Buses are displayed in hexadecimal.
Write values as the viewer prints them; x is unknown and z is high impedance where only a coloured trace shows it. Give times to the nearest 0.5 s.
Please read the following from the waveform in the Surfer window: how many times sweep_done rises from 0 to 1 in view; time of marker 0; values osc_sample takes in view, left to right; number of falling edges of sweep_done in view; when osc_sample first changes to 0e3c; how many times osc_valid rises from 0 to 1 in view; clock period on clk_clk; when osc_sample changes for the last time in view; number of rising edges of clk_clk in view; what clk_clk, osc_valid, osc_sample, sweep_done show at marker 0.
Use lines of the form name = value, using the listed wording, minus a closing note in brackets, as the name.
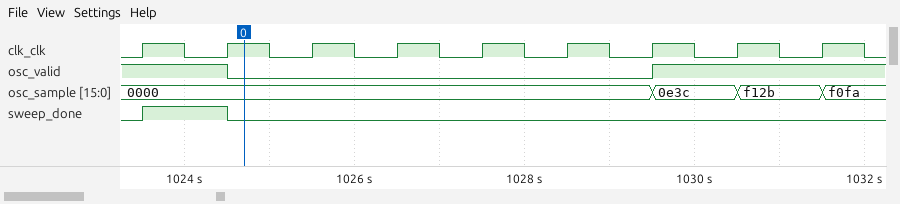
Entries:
how many times sweep_done rises from 0 to 1 in view = 1
time of marker 0 = 1024.5 s
values osc_sample takes in view, left to right = 0000, 0e3c, f12b, f0fa
number of falling edges of sweep_done in view = 1
when osc_sample first changes to 0e3c = 1029.5 s
how many times osc_valid rises from 0 to 1 in view = 1
clock period on clk_clk = 1 s
when osc_sample changes for the last time in view = 1031.5 s
number of rising edges of clk_clk in view = 9
what clk_clk, osc_valid, osc_sample, sweep_done show at marker 0 = clk_clk=1, osc_valid=0, osc_sample=0000, sweep_done=0
